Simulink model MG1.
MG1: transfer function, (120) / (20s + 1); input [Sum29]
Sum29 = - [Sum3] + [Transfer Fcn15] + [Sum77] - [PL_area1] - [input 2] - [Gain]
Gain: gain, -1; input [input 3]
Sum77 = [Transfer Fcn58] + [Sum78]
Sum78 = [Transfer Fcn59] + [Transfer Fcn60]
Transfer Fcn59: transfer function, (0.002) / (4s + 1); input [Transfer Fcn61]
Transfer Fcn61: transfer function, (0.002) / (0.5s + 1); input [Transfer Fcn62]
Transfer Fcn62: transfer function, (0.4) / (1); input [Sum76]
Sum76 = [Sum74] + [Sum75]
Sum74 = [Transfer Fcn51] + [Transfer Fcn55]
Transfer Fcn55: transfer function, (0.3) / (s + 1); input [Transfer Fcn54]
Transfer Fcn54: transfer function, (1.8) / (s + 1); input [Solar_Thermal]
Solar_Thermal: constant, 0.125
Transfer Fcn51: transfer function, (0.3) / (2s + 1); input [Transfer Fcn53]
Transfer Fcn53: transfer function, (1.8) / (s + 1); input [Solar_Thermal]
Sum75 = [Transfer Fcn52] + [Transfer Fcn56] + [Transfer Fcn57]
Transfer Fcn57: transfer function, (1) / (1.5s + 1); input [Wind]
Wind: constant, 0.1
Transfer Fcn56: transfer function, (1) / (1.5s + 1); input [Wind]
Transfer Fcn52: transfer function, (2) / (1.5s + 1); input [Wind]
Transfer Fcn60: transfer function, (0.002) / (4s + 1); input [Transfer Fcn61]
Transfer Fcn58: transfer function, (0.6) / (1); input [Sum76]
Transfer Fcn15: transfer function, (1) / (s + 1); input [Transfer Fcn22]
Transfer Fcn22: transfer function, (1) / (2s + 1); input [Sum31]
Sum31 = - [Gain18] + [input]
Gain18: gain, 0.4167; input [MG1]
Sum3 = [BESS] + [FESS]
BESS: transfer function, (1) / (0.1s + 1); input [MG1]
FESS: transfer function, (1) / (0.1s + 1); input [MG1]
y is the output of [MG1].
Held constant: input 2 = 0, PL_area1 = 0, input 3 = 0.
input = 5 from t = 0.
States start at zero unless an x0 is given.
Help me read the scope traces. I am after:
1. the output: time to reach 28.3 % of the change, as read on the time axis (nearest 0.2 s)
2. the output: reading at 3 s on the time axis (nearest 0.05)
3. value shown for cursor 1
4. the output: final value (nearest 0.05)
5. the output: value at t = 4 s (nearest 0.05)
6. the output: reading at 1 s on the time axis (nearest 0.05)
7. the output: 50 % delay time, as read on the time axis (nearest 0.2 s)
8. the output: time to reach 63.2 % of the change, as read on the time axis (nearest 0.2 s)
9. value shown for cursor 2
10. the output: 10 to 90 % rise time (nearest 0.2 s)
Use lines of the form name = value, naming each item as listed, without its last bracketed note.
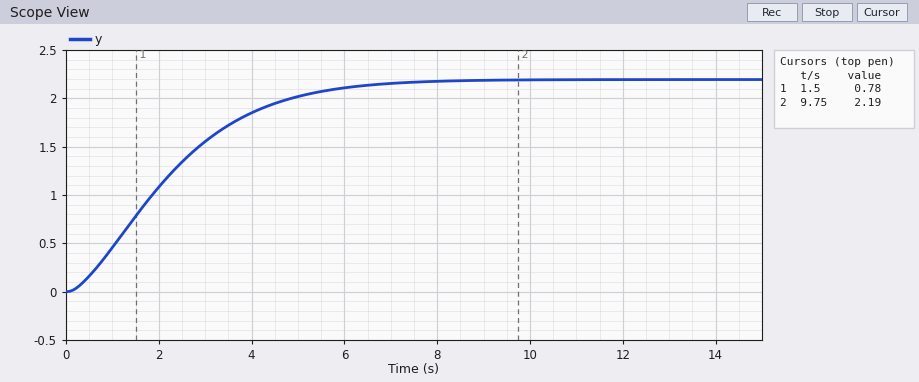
the output: time to reach 28.3 % of the change, as read on the time axis = 1.2 s
the output: reading at 3 s on the time axis = 1.55
value shown for cursor 1 = 0.78
the output: final value = 2.20
the output: value at t = 4 s = 1.85
the output: reading at 1 s on the time axis = 0.45
the output: 50 % delay time, as read on the time axis = 2.0 s
the output: time to reach 63.2 % of the change, as read on the time axis = 2.6 s
value shown for cursor 2 = 2.19
the output: 10 to 90 % rise time = 4.0 s
